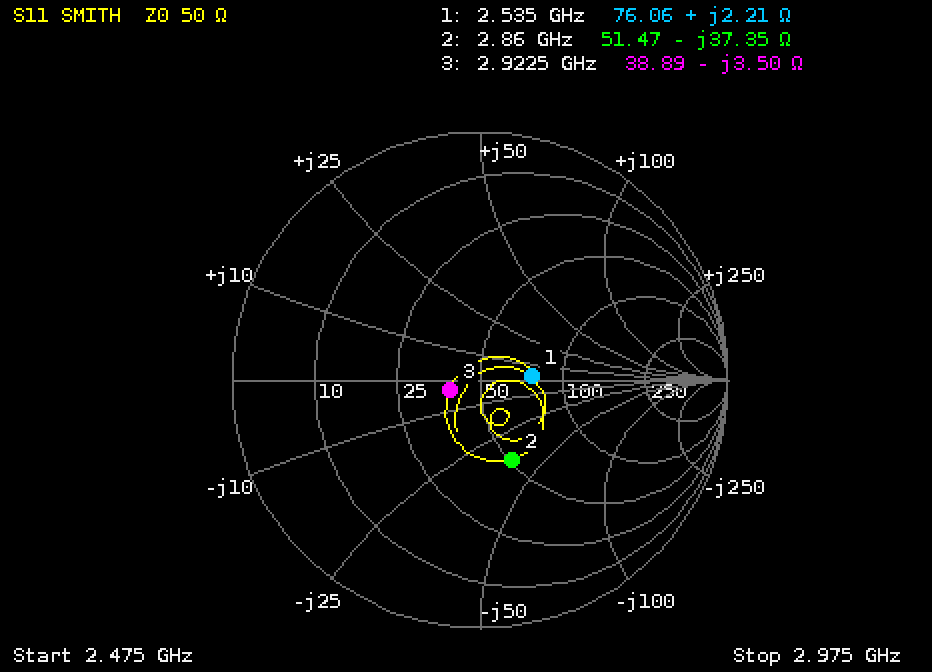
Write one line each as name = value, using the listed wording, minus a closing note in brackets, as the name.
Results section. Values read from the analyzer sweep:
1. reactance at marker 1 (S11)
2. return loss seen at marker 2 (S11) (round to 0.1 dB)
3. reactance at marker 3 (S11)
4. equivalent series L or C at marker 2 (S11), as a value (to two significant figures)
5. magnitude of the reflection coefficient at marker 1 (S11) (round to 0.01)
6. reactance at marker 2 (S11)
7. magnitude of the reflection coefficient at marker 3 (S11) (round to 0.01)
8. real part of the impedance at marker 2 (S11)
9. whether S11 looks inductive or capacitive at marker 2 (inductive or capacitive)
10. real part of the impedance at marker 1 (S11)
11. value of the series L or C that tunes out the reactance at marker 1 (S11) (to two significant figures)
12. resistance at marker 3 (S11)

reactance at marker 1 = +2.21 Ω
return loss seen at marker 2 (S11) = 9.2 dB
reactance at marker 3 = -3.50 Ω
equivalent series L or C at marker 2 (S11), as a value = 1.5 pF
magnitude of the reflection coefficient at marker 1 (S11) = 0.21
reactance at marker 2 = -37.35 Ω
magnitude of the reflection coefficient at marker 3 (S11) = 0.13
real part of the impedance at marker 2 = 51.47 Ω
whether S11 looks inductive or capacitive at marker 2 = capacitive
real part of the impedance at marker 1 = 76.06 Ω
value of the series L or C that tunes out the reactance at marker 1 (S11) = 28 pF
resistance at marker 3 = 38.89 Ω
